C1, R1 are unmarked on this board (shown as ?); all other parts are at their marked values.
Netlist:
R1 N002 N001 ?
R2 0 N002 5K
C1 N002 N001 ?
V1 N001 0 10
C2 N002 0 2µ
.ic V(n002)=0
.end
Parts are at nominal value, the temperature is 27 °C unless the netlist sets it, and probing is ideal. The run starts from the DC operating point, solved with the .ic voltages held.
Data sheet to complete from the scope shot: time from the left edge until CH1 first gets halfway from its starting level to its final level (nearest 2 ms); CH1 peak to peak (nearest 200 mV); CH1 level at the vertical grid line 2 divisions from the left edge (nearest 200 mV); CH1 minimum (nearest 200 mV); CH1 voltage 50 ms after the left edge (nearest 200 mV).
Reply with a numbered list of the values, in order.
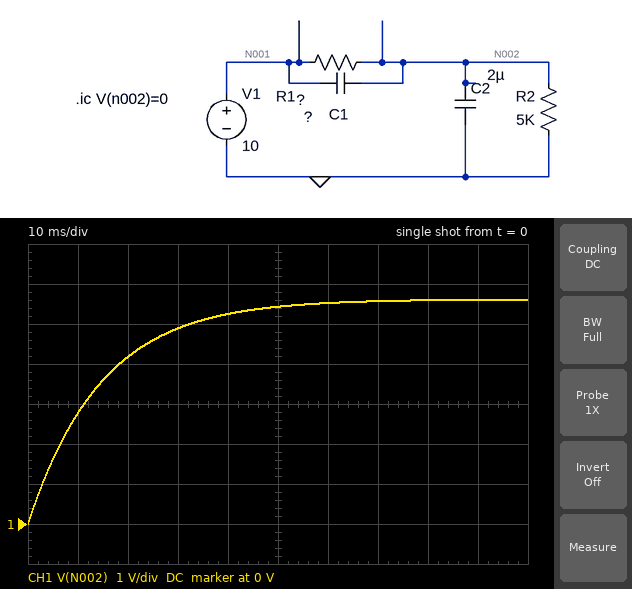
1. 10 ms
2. 5.6 V
3. 4.2 V
4. 0 V
5. 5.4 V
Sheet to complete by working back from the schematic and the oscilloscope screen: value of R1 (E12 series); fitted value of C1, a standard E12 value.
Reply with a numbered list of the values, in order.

1. 3.9 kΩ
2. 4.7 µF
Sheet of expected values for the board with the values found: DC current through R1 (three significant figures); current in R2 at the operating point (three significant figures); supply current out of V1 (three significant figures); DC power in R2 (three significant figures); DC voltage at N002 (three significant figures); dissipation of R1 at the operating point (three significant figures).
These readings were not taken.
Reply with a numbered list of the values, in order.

1. 1.12 mA
2. 1.12 mA
3. 1.12 mA
4. 6.31 mW
5. 5.62 V
6. 4.92 mW
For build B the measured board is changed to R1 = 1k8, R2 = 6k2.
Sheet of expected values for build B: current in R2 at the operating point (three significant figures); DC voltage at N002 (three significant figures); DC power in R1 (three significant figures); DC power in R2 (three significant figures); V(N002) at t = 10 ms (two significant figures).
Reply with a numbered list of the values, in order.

1. 1.25 mA
2. 7.75 V
3. 2.81 mW
4. 9.69 mW
5. 5.1 V
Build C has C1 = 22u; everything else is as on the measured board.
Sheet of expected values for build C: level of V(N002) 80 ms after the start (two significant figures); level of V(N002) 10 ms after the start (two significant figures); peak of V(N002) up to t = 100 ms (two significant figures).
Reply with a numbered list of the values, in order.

1. 4.4 V
2. 970 mV
3. 4.8 V
